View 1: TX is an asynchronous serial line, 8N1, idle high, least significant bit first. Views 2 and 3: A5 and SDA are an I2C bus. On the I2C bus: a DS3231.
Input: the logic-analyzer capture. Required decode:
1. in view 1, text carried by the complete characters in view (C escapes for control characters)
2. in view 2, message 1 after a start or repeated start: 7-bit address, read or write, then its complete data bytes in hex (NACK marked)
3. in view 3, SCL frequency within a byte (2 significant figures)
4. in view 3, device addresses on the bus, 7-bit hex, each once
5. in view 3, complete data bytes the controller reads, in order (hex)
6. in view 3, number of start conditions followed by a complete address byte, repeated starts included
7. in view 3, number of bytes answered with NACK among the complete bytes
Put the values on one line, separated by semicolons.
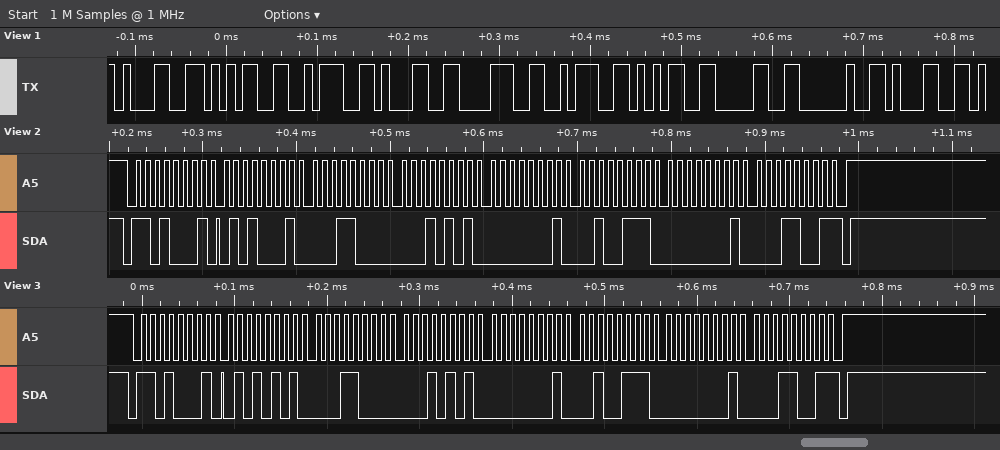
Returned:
"15:18:50 1"; 0x68 read: 51 18 15 01 27 01 19 NACK; 100 kHz; 0x68; 55 18 15 01 27 01 19; 1; 1
